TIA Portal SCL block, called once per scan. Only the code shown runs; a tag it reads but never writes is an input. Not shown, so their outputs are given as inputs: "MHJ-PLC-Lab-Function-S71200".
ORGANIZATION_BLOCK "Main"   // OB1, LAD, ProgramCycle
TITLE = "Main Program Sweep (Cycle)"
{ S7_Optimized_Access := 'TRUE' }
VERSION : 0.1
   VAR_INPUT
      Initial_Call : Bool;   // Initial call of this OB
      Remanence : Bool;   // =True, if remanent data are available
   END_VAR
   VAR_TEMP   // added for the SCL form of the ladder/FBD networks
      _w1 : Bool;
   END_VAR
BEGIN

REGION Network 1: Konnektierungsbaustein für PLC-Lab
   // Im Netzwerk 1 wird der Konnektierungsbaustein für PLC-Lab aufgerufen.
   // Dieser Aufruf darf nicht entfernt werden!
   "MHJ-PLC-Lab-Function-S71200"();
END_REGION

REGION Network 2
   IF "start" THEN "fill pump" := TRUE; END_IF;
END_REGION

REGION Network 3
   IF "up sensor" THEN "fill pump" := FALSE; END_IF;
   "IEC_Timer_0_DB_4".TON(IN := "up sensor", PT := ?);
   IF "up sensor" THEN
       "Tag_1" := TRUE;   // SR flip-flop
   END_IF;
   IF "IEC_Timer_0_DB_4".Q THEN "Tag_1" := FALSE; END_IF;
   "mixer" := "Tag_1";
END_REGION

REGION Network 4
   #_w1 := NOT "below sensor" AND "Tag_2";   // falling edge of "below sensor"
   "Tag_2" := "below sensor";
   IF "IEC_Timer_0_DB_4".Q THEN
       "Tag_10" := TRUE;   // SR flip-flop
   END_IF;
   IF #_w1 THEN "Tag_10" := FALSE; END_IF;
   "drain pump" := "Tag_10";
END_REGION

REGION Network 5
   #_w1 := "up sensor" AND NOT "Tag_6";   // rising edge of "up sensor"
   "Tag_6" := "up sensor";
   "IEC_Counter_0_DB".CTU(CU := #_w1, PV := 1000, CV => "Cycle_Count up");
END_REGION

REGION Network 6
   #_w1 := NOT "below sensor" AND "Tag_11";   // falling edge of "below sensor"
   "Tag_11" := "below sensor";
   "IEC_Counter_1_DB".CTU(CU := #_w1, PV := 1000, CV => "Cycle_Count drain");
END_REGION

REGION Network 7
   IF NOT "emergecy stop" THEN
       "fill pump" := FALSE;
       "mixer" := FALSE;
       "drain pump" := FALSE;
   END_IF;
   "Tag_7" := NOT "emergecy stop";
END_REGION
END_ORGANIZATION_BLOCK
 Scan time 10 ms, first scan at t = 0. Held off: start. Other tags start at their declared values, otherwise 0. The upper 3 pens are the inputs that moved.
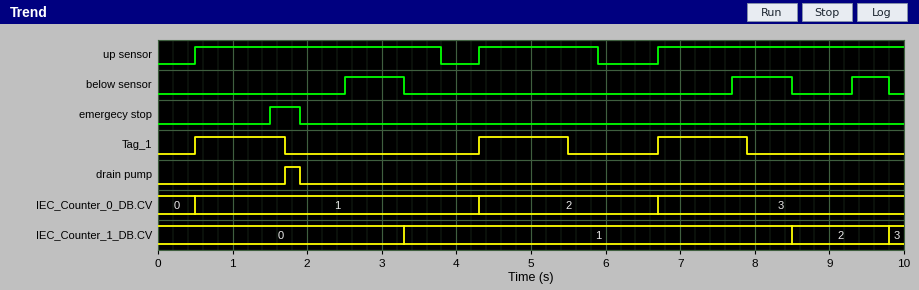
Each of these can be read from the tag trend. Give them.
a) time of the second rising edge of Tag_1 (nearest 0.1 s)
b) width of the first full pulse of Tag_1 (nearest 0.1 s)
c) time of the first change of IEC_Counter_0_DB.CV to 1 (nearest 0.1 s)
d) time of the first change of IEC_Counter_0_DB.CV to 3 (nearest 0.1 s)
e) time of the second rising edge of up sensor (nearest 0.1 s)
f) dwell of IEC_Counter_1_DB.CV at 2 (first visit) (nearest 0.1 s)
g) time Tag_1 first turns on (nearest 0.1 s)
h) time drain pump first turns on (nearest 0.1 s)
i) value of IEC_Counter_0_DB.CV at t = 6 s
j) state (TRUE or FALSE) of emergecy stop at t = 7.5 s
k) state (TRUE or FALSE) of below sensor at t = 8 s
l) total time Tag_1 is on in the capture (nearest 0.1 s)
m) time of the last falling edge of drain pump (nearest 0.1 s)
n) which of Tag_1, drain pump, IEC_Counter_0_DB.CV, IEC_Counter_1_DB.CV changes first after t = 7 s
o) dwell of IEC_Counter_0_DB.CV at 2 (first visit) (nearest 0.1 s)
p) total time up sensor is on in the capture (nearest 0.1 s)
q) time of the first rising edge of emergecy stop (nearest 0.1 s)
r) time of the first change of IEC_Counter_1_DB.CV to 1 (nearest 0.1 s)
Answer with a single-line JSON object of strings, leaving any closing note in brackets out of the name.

{"time of the second rising edge of Tag_1": "4.3 s", "width of the first full pulse of Tag_1": "1.2 s", "time of the first change of IEC_Counter_0_DB.CV to 1": "0.5 s", "time of the first change of IEC_Counter_0_DB.CV to 3": "6.7 s", "time of the second rising edge of up sensor": "4.3 s", "dwell of IEC_Counter_1_DB.CV at 2 (first visit)": "1.3 s", "time Tag_1 first turns on": "0.5 s", "time drain pump first turns on": "1.7 s", "value of IEC_Counter_0_DB.CV at t = 6 s": "2", "state (TRUE or FALSE) of emergecy stop at t = 7.5 s": "FALSE", "state (TRUE or FALSE) of below sensor at t = 8 s": "TRUE", "total time Tag_1 is on in the capture": "3.6 s", "time of the last falling edge of drain pump": "1.9 s", "which of Tag_1, drain pump, IEC_Counter_0_DB.CV, IEC_Counter_1_DB.CV changes first after t = 7 s": "Tag_1", "dwell of IEC_Counter_0_DB.CV at 2 (first visit)": "2.4 s", "total time up sensor is on in the capture": "8.2 s", "time of the first rising edge of emergecy stop": "1.5 s", "time of the first change of IEC_Counter_1_DB.CV to 1": "3.3 s"}
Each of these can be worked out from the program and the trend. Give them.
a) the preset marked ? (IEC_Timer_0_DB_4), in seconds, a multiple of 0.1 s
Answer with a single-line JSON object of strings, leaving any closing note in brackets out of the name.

{"the preset marked ? (IEC_Timer_0_DB_4), in seconds, a multiple of 0.1 s": "1.2 s"}
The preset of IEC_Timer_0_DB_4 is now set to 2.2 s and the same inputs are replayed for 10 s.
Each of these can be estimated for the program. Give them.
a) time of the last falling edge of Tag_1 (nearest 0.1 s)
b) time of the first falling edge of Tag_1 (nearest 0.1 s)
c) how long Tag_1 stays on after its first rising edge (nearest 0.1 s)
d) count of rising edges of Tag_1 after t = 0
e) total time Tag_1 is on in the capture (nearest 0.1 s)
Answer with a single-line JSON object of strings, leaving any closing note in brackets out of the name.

{"time of the last falling edge of Tag_1": "8.9 s", "time of the first falling edge of Tag_1": "2.7 s", "how long Tag_1 stays on after its first rising edge": "2.2 s", "count of rising edges of Tag_1 after t = 0": "2", "total time Tag_1 is on in the capture": "6.8 s"}
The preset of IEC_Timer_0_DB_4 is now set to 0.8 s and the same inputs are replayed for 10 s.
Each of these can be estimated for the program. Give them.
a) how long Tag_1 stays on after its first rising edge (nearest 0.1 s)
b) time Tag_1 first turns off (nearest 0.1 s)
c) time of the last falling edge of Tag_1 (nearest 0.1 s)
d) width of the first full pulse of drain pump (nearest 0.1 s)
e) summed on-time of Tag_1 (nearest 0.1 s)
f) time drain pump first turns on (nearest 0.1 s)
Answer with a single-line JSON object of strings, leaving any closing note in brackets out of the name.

{"how long Tag_1 stays on after its first rising edge": "0.8 s", "time Tag_1 first turns off": "1.3 s", "time of the last falling edge of Tag_1": "7.5 s", "width of the first full pulse of drain pump": "0.4 s", "summed on-time of Tag_1": "2.4 s", "time drain pump first turns on": "1.5 s"}
